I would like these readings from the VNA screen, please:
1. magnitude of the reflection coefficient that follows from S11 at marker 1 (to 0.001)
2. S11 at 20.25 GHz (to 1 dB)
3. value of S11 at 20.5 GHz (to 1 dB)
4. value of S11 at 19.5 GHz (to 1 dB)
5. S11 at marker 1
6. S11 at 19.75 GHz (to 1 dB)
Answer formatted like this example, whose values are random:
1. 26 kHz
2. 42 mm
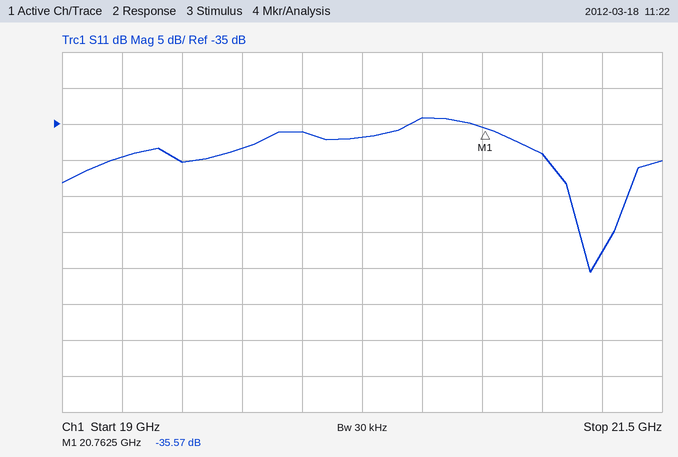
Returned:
1. 0.017
2. -37 dB
3. -34 dB
4. -40 dB
5. -35.57 dB
6. -38 dB
